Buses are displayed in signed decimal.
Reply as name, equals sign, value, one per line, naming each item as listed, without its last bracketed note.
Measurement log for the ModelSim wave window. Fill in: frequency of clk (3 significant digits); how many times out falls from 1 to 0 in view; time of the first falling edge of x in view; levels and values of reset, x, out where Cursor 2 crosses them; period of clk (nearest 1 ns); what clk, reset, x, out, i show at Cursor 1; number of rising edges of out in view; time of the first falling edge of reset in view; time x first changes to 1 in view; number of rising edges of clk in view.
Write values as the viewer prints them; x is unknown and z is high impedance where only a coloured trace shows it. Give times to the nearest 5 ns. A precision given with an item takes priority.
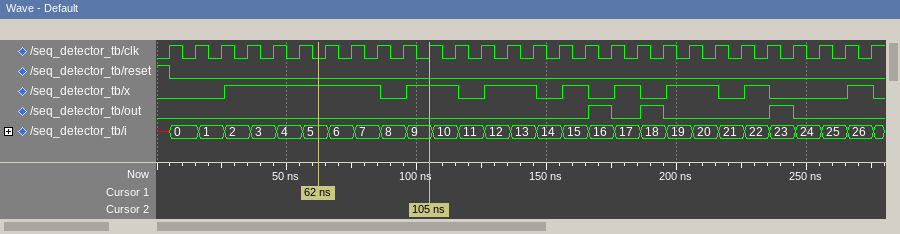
frequency of clk = 100 MHz
how many times out falls from 1 to 0 in view = 3
time of the first falling edge of x in view = 85 ns
levels and values of reset, x, out where Cursor 2 crosses them = reset=0, x=1, out=0
period of clk = 10 ns
what clk, reset, x, out, i show at Cursor 1 = clk=0, reset=0, x=1, out=0, i=5
number of rising edges of out in view = 3
time of the first falling edge of reset in view = 5 ns
time x first changes to 1 in view = 25 ns
number of rising edges of clk in view = 28
